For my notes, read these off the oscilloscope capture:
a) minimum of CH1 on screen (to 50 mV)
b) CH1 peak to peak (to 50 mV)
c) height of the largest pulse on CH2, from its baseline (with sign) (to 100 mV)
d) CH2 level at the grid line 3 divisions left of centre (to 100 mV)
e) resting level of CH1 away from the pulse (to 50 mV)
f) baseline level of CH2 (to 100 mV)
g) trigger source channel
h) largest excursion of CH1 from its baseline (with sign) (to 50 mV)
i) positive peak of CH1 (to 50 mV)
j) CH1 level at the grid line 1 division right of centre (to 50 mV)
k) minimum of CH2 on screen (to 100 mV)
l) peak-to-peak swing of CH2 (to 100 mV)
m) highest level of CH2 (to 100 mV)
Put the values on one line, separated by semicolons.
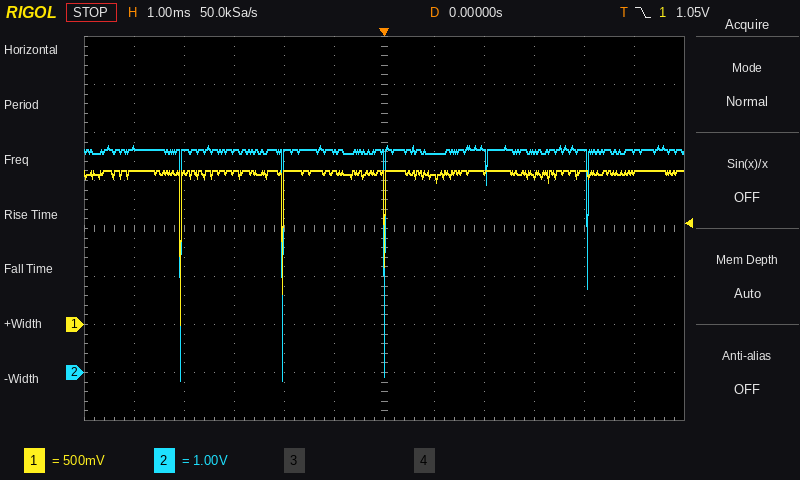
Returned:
0 mV; 1.60 V; -4.8 V; 4.6 V; 1.60 V; 4.6 V; CH1; -1.60 V; 1.60 V; 1.50 V; -200 mV; 4.9 V; 4.7 V
